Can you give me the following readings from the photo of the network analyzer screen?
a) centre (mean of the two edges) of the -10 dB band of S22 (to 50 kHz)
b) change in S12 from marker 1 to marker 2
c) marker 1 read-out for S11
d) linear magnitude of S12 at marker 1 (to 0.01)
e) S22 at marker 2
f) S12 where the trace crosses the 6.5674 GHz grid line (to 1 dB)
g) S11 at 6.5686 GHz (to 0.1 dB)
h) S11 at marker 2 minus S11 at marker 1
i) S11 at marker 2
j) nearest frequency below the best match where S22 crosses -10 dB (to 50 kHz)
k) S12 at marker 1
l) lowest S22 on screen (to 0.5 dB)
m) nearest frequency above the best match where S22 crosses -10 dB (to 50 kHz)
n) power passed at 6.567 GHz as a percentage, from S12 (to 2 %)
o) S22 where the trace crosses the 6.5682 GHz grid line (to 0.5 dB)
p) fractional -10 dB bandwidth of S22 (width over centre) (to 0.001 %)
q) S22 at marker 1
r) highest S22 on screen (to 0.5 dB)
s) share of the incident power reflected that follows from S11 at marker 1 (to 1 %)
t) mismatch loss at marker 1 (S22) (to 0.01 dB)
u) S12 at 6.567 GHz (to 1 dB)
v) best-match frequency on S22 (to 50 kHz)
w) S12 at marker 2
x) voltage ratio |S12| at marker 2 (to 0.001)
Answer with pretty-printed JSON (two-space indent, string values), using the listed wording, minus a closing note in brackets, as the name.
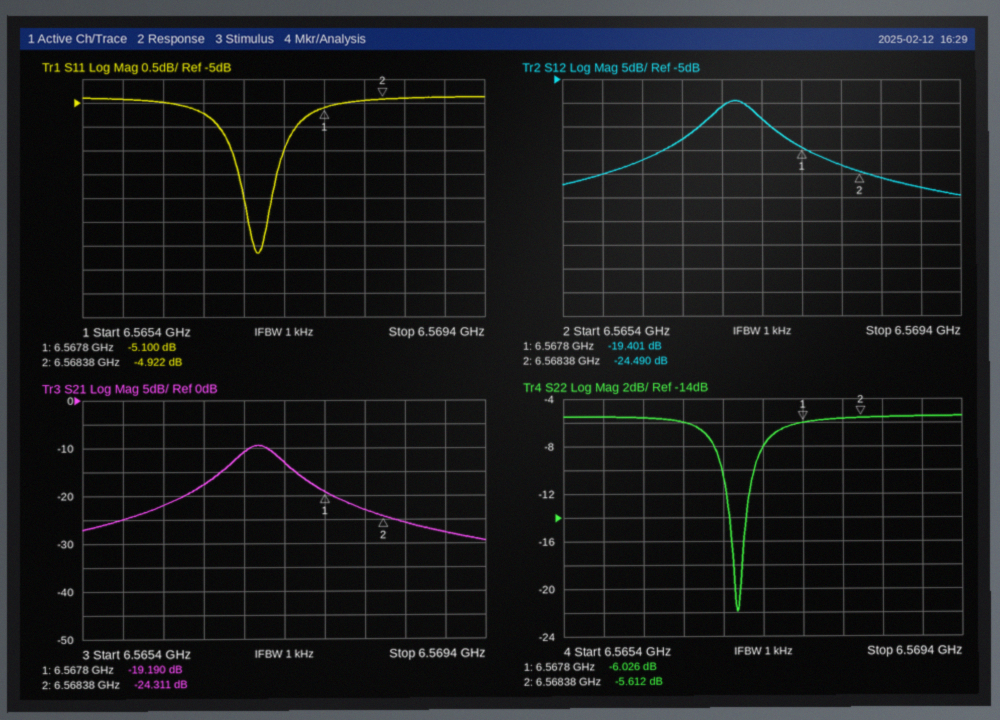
{
  "centre (mean of the two edges) of the -10 dB band of S22": "6.56715 GHz",
  "change in S12 from marker 1 to marker 2": "-5.089 dB",
  "marker 1 read-out for S11": "-5.100 dB",
  "linear magnitude of S12 at marker 1": "0.11",
  "S22 at marker 2": "-5.612 dB",
  "S12 where the trace crosses the 6.5674 GHz grid line": "-13 dB",
  "S11 at 6.5686 GHz": "-4.9 dB",
  "S11 at marker 2 minus S11 at marker 1": "0.178 dB",
  "S11 at marker 2": "-4.922 dB",
  "nearest frequency below the best match where S22 crosses -10 dB": "6.56700 GHz",
  "S12 at marker 1": "-19.401 dB",
  "lowest S22 on screen": "-22.0 dB",
  "nearest frequency above the best match where S22 crosses -10 dB": "6.56730 GHz",
  "power passed at 6.567 GHz as a percentage, from S12": "8 %",
  "S22 where the trace crosses the 6.5682 GHz grid line": "-5.5 dB",
  "fractional -10 dB bandwidth of S22 (width over centre)": "0.005 %",
  "S22 at marker 1": "-6.026 dB",
  "highest S22 on screen": "-5.5 dB",
  "share of the incident power reflected that follows from S11 at marker 1": "31 %",
  "mismatch loss at marker 1 (S22)": "1.25 dB",
  "S12 at 6.567 GHz": "-11 dB",
  "best-match frequency on S22": "6.56715 GHz",
  "S12 at marker 2": "-24.490 dB",
  "voltage ratio |S12| at marker 2": "0.060"
}
